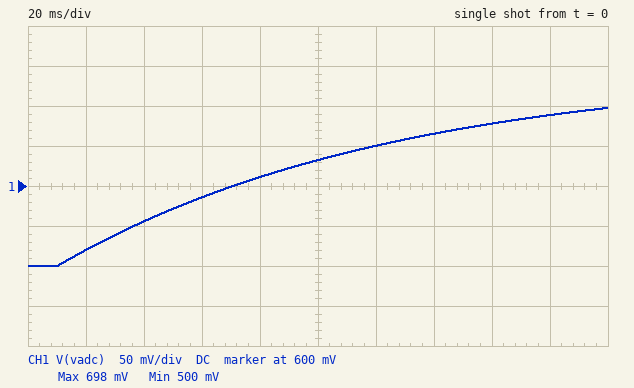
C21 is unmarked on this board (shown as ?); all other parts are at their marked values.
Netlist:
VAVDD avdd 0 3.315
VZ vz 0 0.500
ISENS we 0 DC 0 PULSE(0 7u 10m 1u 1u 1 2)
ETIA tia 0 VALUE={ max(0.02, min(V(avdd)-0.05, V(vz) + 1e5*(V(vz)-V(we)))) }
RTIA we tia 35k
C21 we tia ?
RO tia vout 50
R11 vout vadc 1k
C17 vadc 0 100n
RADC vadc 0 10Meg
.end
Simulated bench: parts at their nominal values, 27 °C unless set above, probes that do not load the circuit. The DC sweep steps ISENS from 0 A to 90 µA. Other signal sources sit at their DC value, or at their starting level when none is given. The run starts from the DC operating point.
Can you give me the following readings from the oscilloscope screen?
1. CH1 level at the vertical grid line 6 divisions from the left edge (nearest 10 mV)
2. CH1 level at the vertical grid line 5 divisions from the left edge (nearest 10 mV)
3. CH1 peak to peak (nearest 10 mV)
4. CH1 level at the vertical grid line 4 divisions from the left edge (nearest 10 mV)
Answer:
650 mV
630 mV
200 mV
610 mV
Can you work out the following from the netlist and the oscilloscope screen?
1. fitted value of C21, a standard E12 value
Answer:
3.3 µF
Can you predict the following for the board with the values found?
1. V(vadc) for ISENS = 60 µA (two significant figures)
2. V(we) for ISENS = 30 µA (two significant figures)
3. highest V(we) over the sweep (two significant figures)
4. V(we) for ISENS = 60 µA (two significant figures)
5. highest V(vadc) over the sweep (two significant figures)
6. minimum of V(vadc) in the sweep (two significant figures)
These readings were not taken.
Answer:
2.6 V
500 mV
500 mV
500 mV
3.3 V
500 mV
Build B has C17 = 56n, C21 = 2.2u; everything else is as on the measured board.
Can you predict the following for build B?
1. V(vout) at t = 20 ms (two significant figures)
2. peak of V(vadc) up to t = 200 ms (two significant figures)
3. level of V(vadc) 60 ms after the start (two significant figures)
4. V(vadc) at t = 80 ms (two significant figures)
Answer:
530 mV
720 mV
620 mV
650 mV
